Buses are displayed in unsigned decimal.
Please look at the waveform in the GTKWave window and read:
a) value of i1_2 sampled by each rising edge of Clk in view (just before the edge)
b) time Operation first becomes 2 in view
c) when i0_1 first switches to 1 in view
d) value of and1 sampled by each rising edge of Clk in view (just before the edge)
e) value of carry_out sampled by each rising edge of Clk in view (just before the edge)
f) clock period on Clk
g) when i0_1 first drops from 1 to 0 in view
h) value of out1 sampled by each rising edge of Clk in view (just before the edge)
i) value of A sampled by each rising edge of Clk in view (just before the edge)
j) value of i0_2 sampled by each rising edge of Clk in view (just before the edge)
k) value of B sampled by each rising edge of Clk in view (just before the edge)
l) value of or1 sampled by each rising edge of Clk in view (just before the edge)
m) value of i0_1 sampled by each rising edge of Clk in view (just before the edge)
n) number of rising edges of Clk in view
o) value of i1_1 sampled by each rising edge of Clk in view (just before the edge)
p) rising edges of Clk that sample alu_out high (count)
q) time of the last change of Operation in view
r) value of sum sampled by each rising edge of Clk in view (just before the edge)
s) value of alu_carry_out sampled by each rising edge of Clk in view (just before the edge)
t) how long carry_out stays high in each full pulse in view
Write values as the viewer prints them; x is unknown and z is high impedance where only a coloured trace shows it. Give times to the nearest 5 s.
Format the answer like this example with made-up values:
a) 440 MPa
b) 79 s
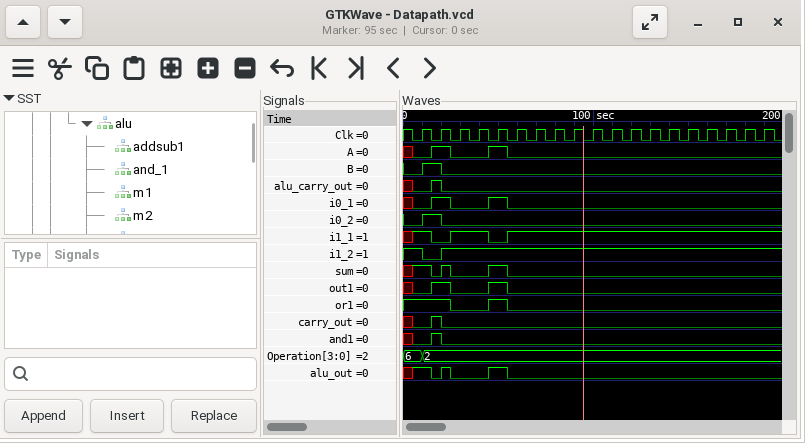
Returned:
a) 1 0 1 1 1 1 1 1 1 1 1 1 1 1 1 1 1 1 1
b) 10 s
c) 15 s
d) 0 1 0 0 0 0 0 0 0 0 0 0 0 0 0 0 0 0 0
e) 0 1 0 0 0 0 0 0 0 0 0 0 0 0 0 0 0 0 0
f) 10 s
g) 25 s
h) 0 1 0 0 1 0 0 0 0 0 0 0 0 0 0 0 0 0 0
i) 0 1 0 0 1 0 0 0 0 0 0 0 0 0 0 0 0 0 0
j) 0 1 0 0 0 0 0 0 0 0 0 0 0 0 0 0 0 0 0
k) 0 1 0 0 0 0 0 0 0 0 0 0 0 0 0 0 0 0 0
l) 1 1 0 0 1 0 0 0 0 0 0 0 0 0 0 0 0 0 0
m) 0 1 0 0 1 0 0 0 0 0 0 0 0 0 0 0 0 0 0
n) 19
o) 1 0 1 1 0 1 1 1 1 1 1 1 1 1 1 1 1 1 1
p) 2
q) 10 s
r) 1 0 0 0 1 0 0 0 0 0 0 0 0 0 0 0 0 0 0
s) 0 1 0 0 0 0 0 0 0 0 0 0 0 0 0 0 0 0 0
t) 5 s
